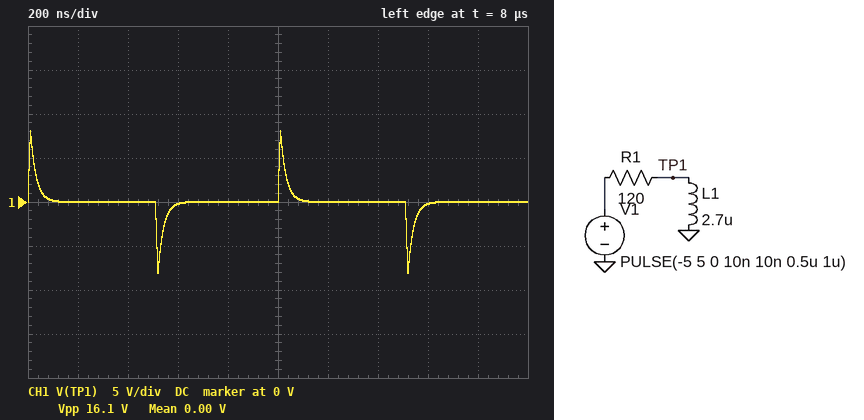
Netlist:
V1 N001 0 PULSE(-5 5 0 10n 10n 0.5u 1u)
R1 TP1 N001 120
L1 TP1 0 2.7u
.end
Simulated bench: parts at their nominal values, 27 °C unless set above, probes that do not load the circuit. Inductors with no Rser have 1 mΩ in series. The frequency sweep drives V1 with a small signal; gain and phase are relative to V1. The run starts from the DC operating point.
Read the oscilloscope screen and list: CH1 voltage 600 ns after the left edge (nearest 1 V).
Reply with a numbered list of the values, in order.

1. 0 V
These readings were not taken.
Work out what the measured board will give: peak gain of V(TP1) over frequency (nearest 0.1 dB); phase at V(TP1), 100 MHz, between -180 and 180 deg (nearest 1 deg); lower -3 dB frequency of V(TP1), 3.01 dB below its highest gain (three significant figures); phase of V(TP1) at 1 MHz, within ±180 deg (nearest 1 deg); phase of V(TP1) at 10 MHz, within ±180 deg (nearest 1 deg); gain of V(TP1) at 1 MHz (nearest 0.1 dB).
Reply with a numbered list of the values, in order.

1. 0 dB
2. 4 deg
3. 7.07 MHz
4. 82 deg
5. 35 deg
6. -17.1 dB
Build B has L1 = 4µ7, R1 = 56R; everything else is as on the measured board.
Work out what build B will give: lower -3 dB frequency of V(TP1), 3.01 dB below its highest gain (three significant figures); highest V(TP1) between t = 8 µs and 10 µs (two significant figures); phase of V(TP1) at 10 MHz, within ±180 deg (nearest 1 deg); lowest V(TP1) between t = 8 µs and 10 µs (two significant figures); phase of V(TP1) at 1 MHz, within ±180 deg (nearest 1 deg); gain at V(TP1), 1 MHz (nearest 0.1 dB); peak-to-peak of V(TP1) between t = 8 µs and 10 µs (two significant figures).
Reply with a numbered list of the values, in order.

1. 1.90 MHz
2. 9.4 V
3. 11 deg
4. -9.4 V
5. 62 deg
6. -6.6 dB
7. 19 V
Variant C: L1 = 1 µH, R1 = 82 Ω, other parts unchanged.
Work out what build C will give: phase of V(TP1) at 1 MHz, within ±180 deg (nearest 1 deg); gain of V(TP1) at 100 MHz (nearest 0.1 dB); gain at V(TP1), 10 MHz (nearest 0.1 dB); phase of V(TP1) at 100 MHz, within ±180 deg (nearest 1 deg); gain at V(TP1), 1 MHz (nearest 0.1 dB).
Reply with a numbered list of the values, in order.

1. 86 deg
2. -0.1 dB
3. -4.3 dB
4. 7 deg
5. -22.3 dB
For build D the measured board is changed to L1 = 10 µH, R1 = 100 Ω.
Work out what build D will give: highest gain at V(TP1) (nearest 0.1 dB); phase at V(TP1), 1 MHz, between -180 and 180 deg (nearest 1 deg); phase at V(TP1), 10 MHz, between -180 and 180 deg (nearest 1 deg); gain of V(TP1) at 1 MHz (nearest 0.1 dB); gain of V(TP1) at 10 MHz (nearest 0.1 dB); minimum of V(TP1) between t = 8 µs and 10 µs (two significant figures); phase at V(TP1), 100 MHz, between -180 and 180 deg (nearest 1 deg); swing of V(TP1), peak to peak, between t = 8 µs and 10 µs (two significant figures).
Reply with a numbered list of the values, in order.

1. 0 dB
2. 58 deg
3. 9 deg
4. -5.5 dB
5. -0.1 dB
6. -9.5 V
7. 1 deg
8. 19 V
